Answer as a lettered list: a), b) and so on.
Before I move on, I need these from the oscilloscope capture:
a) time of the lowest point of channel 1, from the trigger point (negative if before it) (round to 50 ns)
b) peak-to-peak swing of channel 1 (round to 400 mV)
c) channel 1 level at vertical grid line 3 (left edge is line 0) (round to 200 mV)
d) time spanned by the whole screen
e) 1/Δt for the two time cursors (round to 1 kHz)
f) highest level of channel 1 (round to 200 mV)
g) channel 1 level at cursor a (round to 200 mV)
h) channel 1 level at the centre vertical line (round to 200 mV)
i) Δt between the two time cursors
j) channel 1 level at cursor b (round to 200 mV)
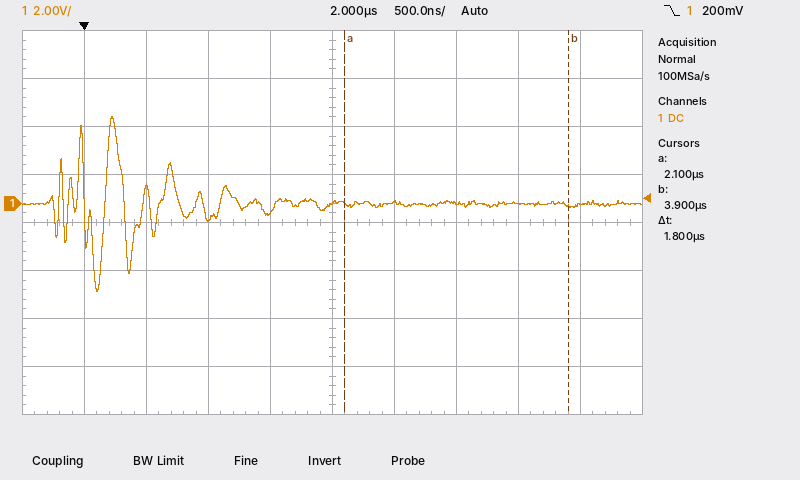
a) +100 ns
b) 7.2 V
c) -600 mV
d) 5 µs
e) 556 kHz
f) 3.6 V
g) 0.0 V
h) 0.0 V
i) 1.8 µs
j) -200 mV
